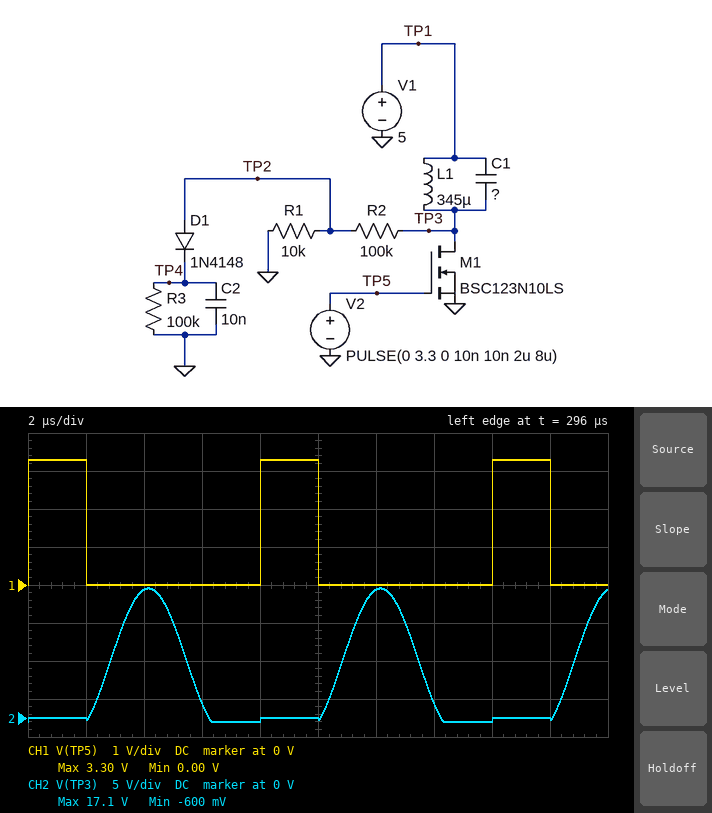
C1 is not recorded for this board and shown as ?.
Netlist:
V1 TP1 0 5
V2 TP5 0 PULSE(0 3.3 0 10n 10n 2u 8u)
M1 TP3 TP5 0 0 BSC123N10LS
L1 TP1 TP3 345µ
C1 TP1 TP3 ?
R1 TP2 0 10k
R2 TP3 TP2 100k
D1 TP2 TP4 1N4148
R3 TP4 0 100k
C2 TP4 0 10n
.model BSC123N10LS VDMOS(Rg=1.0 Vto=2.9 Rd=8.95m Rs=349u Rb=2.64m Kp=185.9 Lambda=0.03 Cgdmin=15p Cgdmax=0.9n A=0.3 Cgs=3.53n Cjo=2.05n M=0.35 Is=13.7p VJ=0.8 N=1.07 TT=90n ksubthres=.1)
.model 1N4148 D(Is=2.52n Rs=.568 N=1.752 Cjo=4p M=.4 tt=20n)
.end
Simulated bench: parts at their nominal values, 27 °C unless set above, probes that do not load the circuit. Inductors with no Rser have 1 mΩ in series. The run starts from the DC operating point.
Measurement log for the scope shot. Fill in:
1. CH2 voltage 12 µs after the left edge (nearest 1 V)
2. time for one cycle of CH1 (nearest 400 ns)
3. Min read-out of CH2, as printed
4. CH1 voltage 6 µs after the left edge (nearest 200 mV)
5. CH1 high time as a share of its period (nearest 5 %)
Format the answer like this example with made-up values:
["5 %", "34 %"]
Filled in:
["17 V", "8.0 µs", "-600 mV", "0 V", "25 %"]
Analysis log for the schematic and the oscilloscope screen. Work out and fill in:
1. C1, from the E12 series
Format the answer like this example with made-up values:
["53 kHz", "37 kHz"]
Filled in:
["1.8 nF"]
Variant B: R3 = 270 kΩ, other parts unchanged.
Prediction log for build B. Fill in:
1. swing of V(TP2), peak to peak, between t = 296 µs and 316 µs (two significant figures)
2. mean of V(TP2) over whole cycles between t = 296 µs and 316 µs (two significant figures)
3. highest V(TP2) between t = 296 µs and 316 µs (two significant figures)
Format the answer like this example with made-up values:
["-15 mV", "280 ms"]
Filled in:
["1.1 V", "370 mV", "1.0 V"]
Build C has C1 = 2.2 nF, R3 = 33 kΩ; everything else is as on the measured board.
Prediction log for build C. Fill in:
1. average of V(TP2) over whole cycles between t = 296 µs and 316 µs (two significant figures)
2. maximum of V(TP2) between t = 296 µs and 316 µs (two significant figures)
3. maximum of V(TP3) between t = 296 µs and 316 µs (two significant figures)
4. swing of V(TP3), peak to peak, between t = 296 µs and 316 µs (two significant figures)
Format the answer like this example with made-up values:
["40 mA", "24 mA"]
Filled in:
["330 mV", "810 mV", "15 V", "16 V"]
